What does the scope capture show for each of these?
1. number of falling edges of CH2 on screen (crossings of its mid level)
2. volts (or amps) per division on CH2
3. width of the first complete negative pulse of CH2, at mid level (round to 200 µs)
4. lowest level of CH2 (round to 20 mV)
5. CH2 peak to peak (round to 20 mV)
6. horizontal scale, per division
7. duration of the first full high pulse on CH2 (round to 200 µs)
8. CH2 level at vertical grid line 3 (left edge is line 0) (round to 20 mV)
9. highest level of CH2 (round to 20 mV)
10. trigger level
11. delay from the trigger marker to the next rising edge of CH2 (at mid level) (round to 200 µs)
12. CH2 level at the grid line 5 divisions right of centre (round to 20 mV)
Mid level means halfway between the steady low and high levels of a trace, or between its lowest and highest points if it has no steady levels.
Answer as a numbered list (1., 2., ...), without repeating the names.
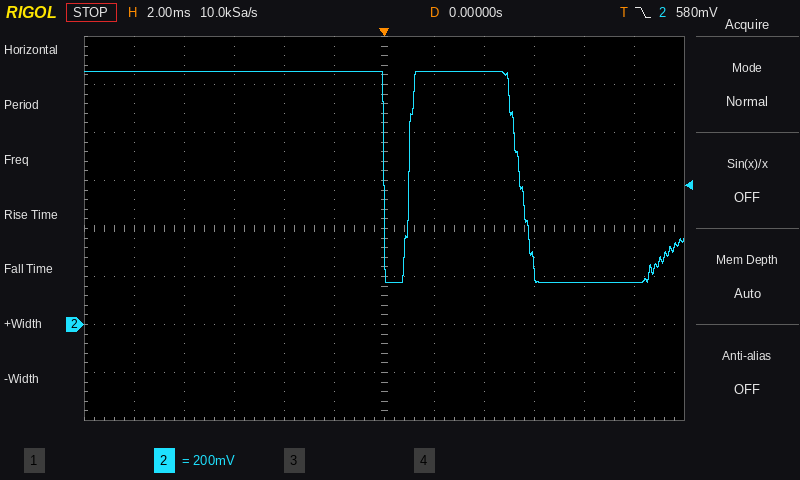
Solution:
1. 2
2. 200 mV
3. 1.0 ms
4. 180 mV
5. 880 mV
6. 2 ms
7. 4.4 ms
8. 1.06 V
9. 1.06 V
10. 580 mV
11. 1.0 ms
12. 180 mV
